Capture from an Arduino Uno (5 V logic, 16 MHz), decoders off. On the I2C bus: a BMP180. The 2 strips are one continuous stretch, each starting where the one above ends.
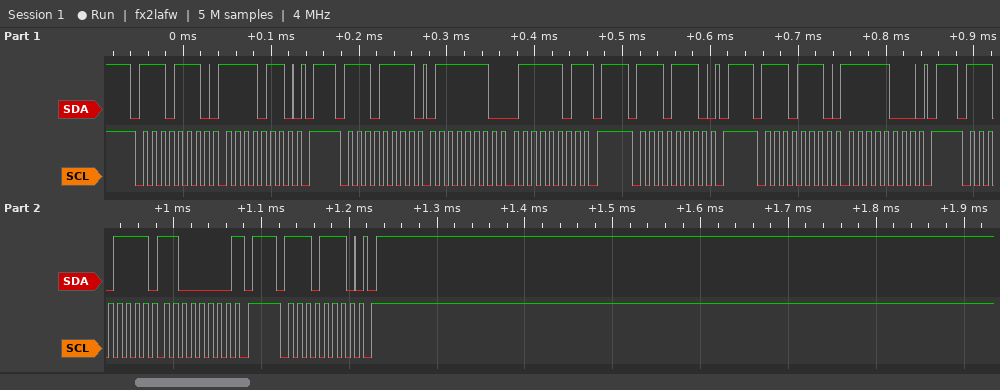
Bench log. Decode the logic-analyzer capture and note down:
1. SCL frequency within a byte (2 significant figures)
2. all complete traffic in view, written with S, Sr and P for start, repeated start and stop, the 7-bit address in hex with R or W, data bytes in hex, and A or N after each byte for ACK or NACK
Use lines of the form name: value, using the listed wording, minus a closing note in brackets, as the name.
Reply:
SCL frequency within a byte: 100 kHz
all complete traffic in view, written with S, Sr and P for start, repeated start and stop, the 7-bit address in hex with R or W, data bytes in hex, and A or N after each byte for ACK or NACK: S 77W A F6 A P S 77R A 7E A 7D N P S 77W A P S 77W A F8 A P S 77R A C0 N P S 77W A P
